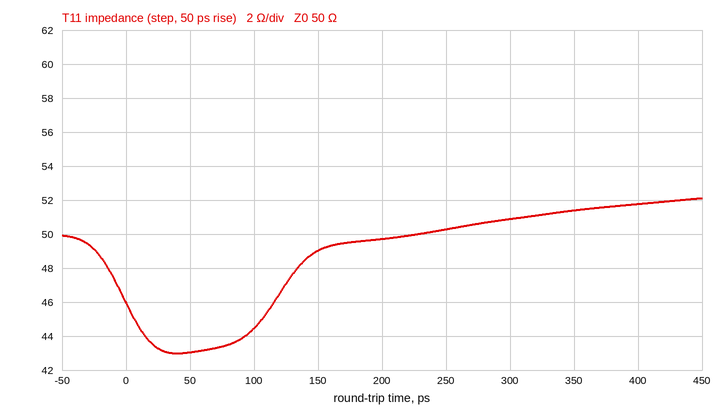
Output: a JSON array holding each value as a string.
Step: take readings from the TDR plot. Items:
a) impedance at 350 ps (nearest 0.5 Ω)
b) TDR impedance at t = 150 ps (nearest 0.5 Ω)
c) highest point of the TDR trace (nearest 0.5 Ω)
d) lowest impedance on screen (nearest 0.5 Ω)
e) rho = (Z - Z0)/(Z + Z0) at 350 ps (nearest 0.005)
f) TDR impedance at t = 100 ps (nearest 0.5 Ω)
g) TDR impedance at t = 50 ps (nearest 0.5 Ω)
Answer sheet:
["51.5 Ω", "49.0 Ω", "52.0 Ω", "43.0 Ω", "+0.015", "44.5 Ω", "43.0 Ω"]
